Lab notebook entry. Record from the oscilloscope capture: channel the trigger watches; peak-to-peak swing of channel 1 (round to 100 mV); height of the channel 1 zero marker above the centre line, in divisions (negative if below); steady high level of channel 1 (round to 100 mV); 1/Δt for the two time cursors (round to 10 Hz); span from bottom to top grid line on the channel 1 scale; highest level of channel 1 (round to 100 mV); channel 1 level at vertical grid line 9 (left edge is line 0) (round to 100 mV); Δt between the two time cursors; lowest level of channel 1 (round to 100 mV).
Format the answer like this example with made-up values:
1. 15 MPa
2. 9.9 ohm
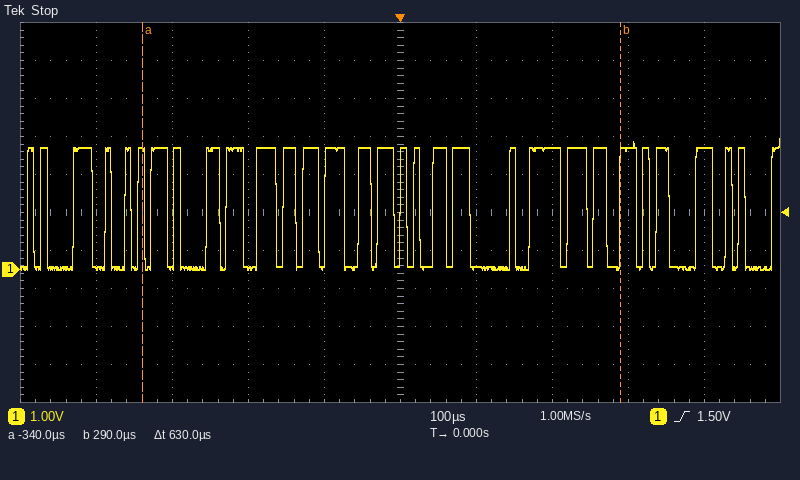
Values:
1. channel 1
2. 3.4 V
3. -1.5 div
4. 3.2 V
5. 1.59 kHz
6. 10 V
7. 3.4 V
8. 3.2 V
9. 630 µs
10. 0.0 V
